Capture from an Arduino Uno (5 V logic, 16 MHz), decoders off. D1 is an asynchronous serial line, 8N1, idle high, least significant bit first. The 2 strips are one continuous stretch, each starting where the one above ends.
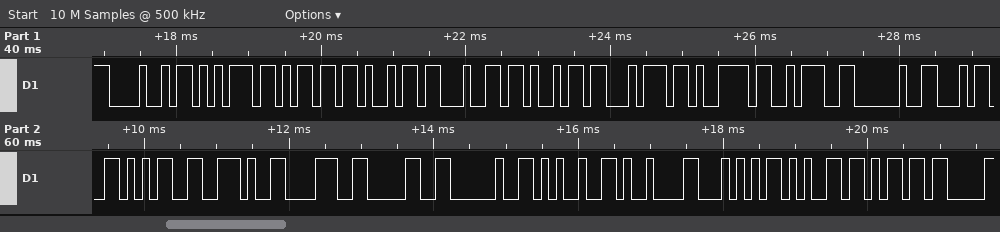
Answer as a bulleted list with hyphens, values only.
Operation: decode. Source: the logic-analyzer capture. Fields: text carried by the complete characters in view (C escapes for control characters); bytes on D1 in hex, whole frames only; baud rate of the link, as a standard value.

- "Humidity: 45.80 %\tTem"
- 48 75 6D 69 64 69 74 79 3A 20 34 35 2E 38 30 20 25 09 54 65 6D
- 9600 baud
